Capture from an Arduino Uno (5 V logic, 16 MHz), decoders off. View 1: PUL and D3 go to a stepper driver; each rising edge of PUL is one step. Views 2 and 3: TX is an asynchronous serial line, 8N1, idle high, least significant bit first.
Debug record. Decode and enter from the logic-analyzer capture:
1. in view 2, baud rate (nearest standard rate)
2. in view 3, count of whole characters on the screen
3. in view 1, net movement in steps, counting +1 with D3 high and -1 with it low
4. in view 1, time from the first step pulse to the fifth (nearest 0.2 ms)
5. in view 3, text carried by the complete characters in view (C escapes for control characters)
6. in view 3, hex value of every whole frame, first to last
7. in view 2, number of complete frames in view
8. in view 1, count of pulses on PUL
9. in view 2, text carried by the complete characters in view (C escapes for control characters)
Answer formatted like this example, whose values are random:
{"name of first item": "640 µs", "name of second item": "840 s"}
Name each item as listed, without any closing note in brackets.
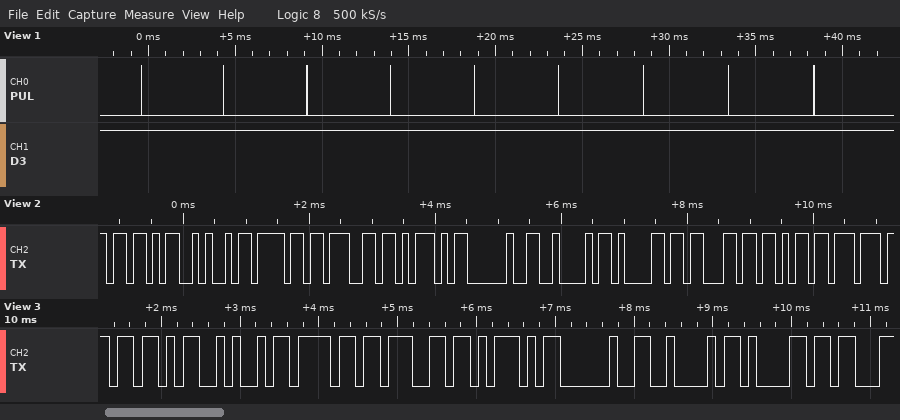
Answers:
{"in view 2, baud rate": "9600 baud", "in view 3, count of whole characters on the screen": "8", "in view 1, net movement in steps, counting +1 with D3 high and -1 with it low": "+9", "in view 1, time from the first step pulse to the fifth": "19.2 ms", "in view 3, text carried by the complete characters in view": "\"[Jog] Ba\"", "in view 3, hex value of every whole frame, first to last": "5B 4A 6F 67 5D 20 42 61", "in view 2, number of complete frames in view": "11", "in view 1, count of pulses on PUL": "9", "in view 2, text carried by the complete characters in view": "\"[Jog] Backw\""}
